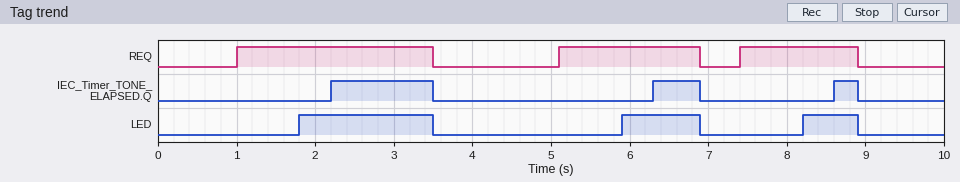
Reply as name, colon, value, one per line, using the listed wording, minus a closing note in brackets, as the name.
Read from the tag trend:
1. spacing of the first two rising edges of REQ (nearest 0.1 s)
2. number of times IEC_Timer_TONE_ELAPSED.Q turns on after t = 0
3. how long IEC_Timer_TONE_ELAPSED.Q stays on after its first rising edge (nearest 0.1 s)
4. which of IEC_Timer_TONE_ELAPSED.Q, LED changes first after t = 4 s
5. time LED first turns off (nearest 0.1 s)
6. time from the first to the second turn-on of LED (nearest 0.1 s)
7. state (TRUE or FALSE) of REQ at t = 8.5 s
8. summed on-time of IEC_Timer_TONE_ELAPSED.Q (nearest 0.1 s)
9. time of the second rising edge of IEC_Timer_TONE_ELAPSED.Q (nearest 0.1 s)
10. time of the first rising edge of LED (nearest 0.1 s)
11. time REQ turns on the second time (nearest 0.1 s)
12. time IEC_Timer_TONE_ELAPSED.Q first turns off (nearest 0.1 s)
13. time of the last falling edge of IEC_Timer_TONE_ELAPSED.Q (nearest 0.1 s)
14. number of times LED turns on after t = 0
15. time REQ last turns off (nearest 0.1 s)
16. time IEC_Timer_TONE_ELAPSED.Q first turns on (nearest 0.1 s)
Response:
spacing of the first two rising edges of REQ: 4.1 s
number of times IEC_Timer_TONE_ELAPSED.Q turns on after t = 0: 3
how long IEC_Timer_TONE_ELAPSED.Q stays on after its first rising edge: 1.3 s
which of IEC_Timer_TONE_ELAPSED.Q, LED changes first after t = 4 s: LED
time LED first turns off: 3.5 s
time from the first to the second turn-on of LED: 4.1 s
state (TRUE or FALSE) of REQ at t = 8.5 s: TRUE
summed on-time of IEC_Timer_TONE_ELAPSED.Q: 2.2 s
time of the second rising edge of IEC_Timer_TONE_ELAPSED.Q: 6.3 s
time of the first rising edge of LED: 1.8 s
time REQ turns on the second time: 5.1 s
time IEC_Timer_TONE_ELAPSED.Q first turns off: 3.5 s
time of the last falling edge of IEC_Timer_TONE_ELAPSED.Q: 8.9 s
number of times LED turns on after t = 0: 3
time REQ last turns off: 8.9 s
time IEC_Timer_TONE_ELAPSED.Q first turns on: 2.2 s
